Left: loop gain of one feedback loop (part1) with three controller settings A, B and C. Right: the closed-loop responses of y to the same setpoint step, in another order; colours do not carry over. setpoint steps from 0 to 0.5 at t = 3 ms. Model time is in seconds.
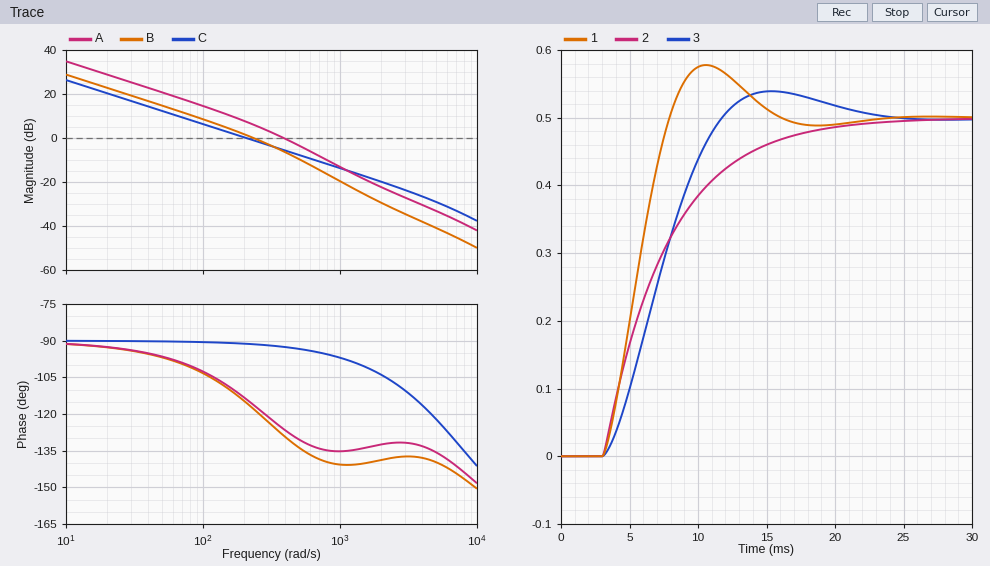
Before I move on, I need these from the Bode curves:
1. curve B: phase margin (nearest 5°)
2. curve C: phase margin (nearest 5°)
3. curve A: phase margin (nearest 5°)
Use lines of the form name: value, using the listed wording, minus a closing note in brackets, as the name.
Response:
curve B: phase margin: 60°
curve C: phase margin: 90°
curve A: phase margin: 55°
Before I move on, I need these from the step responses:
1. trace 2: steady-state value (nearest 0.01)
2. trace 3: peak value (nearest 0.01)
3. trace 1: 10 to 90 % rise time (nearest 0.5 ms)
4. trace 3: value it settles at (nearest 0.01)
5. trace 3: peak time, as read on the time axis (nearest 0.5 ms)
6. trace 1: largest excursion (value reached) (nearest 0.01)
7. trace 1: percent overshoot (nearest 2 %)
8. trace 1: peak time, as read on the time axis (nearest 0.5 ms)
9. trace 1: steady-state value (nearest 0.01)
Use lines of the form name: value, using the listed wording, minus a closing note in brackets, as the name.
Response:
trace 2: steady-state value: 0.50
trace 3: peak value: 0.54
trace 1: 10 to 90 % rise time: 3.5 ms
trace 3: value it settles at: 0.50
trace 3: peak time, as read on the time axis: 15.5 ms
trace 1: largest excursion (value reached): 0.58
trace 1: percent overshoot: 16 %
trace 1: peak time, as read on the time axis: 10.5 ms
trace 1: steady-state value: 0.50
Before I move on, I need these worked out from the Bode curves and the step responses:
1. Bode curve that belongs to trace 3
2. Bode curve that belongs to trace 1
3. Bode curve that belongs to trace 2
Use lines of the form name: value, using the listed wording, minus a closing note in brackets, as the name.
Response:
Bode curve that belongs to trace 3: B
Bode curve that belongs to trace 1: A
Bode curve that belongs to trace 2: C
